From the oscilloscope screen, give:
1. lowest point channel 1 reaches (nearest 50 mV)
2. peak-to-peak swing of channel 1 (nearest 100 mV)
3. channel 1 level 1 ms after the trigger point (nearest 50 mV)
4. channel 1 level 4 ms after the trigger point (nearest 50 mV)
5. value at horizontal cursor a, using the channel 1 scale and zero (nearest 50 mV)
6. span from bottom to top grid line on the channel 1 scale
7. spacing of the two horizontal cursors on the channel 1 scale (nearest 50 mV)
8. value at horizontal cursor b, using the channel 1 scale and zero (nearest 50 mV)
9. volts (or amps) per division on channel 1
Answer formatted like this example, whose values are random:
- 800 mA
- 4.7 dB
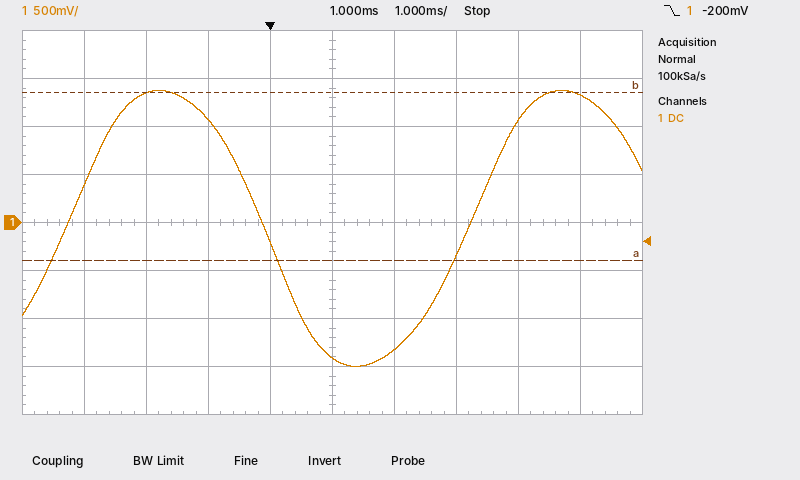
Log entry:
- -1.50 V
- 2.90 V
- -1.40 V
- 1.05 V
- -400 mV
- 4 V
- 1.75 V
- 1.35 V
- 500 mV
